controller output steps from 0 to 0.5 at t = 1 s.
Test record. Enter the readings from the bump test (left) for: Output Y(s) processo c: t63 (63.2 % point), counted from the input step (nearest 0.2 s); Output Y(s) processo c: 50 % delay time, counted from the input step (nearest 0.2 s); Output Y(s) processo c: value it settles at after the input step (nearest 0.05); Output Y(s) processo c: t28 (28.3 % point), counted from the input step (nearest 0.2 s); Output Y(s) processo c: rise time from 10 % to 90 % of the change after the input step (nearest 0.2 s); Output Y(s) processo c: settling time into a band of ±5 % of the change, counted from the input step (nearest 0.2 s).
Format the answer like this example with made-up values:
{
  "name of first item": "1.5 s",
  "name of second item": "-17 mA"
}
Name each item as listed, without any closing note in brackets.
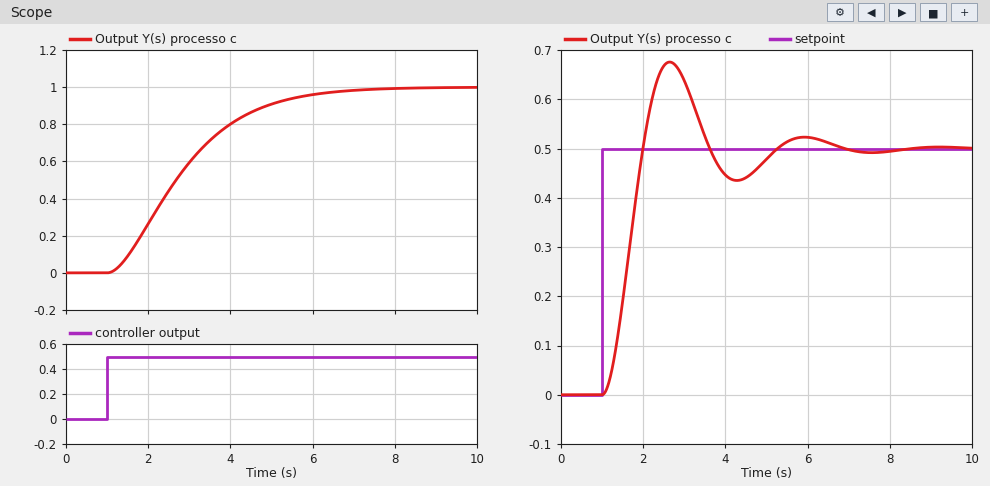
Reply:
{
  "Output Y(s) processo c: t63 (63.2 % point), counted from the input step": "2.2 s",
  "Output Y(s) processo c: 50 % delay time, counted from the input step": "1.6 s",
  "Output Y(s) processo c: value it settles at after the input step": "1.00",
  "Output Y(s) processo c: t28 (28.3 % point), counted from the input step": "1.0 s",
  "Output Y(s) processo c: rise time from 10 % to 90 % of the change after the input step": "3.4 s",
  "Output Y(s) processo c: settling time into a band of ±5 % of the change, counted from the input step": "4.8 s"
}
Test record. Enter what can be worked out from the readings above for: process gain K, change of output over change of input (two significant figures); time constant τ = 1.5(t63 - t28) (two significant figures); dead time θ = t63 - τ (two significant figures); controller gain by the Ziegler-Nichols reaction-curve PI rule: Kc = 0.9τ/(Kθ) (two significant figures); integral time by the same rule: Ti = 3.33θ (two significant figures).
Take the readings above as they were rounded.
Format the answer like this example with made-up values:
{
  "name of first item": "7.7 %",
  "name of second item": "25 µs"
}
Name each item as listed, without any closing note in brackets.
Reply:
{
  "process gain K, change of output over change of input": "2.0",
  "time constant τ = 1.5(t63 - t28)": "1.8 s",
  "dead time θ = t63 - τ": "0.40 s",
  "controller gain by the Ziegler-Nichols reaction-curve PI rule: Kc = 0.9τ/(Kθ)": "2.0",
  "integral time by the same rule: Ti = 3.33θ": "1.3 s"
}
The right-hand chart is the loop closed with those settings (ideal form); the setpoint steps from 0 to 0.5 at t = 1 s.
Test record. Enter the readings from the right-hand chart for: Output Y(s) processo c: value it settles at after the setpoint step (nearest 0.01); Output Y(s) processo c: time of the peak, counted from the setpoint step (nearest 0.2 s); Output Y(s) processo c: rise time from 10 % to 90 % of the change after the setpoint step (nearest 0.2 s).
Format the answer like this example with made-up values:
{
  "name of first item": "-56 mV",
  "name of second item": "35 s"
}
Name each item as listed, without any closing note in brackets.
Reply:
{
  "Output Y(s) processo c: value it settles at after the setpoint step": "0.50",
  "Output Y(s) processo c: time of the peak, counted from the setpoint step": "1.6 s",
  "Output Y(s) processo c: rise time from 10 % to 90 % of the change after the setpoint step": "0.6 s"
}
